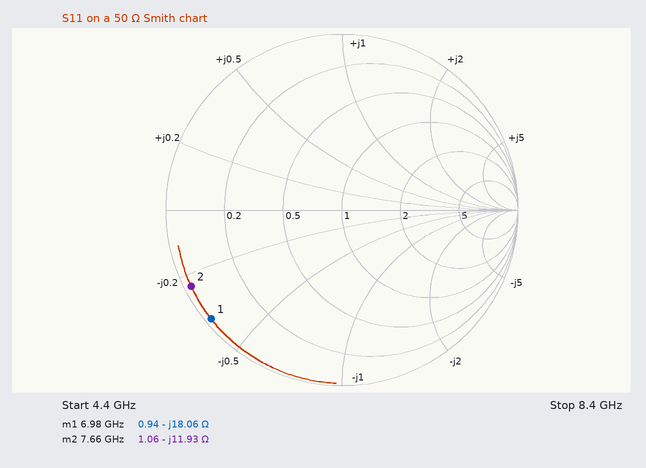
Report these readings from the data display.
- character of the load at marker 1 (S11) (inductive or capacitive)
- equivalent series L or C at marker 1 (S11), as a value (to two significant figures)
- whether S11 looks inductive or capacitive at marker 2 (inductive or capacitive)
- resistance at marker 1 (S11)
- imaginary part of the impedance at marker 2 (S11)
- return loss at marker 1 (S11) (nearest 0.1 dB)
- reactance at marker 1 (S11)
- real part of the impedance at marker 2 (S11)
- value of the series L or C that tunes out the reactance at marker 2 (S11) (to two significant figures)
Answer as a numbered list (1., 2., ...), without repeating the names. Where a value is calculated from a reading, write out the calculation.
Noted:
1. capacitive
2. C = 1/(2π × 6.98 GHz × 18.06 Ω) ≈ 1.3 pF
3. capacitive
4. 0.94 Ω
5. -11.93 Ω
6. 0.3 dB
7. -18.06 Ω
8. 1.06 Ω
9. L = 11.93 Ω/(2π × 7.66 GHz) ≈ 248 pH, so 250 pH to two significant figures
